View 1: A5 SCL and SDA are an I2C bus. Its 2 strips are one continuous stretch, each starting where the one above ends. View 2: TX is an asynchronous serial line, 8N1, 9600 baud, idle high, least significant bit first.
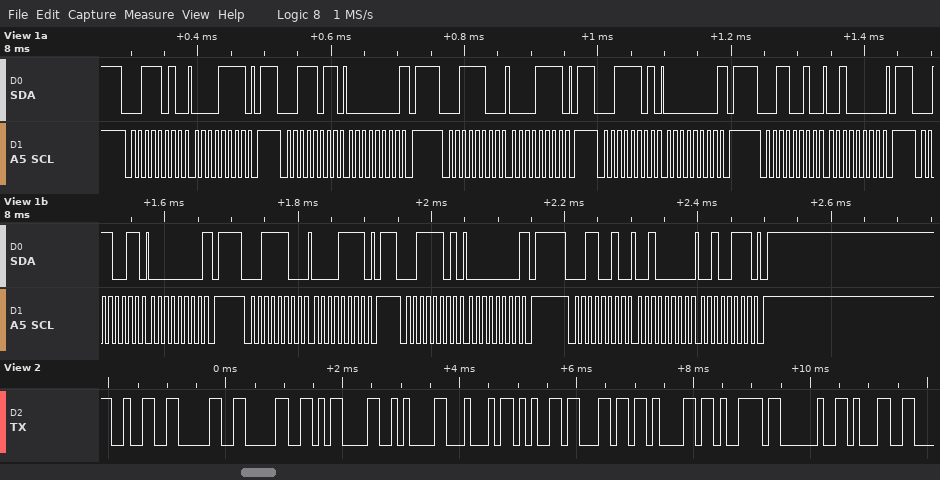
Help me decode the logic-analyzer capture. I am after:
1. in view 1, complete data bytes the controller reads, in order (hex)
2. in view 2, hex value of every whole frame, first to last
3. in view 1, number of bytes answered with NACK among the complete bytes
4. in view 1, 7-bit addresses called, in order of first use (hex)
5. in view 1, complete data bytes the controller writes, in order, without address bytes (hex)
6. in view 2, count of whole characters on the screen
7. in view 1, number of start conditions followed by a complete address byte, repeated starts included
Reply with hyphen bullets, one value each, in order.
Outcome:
- 00 00 00 00
- 32 30 30 0D 0A 44 65 6C 61 79 20 31
- 4
- 0x1D 0x1E 0x19
- 0F 0F 20 0F 20 27
- 12
- 9
